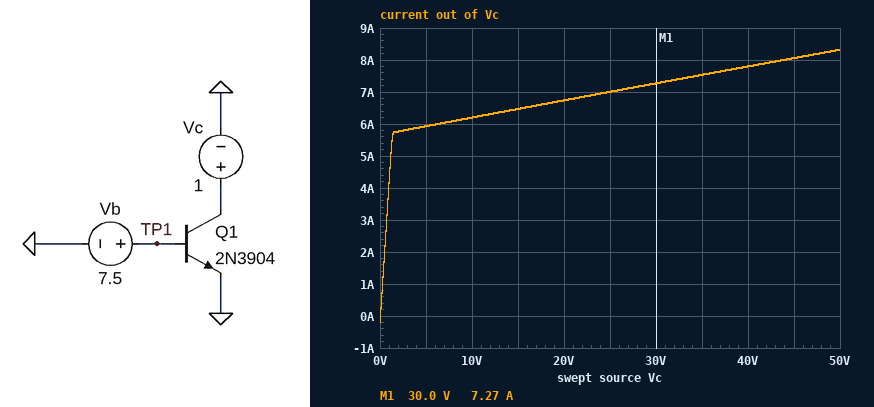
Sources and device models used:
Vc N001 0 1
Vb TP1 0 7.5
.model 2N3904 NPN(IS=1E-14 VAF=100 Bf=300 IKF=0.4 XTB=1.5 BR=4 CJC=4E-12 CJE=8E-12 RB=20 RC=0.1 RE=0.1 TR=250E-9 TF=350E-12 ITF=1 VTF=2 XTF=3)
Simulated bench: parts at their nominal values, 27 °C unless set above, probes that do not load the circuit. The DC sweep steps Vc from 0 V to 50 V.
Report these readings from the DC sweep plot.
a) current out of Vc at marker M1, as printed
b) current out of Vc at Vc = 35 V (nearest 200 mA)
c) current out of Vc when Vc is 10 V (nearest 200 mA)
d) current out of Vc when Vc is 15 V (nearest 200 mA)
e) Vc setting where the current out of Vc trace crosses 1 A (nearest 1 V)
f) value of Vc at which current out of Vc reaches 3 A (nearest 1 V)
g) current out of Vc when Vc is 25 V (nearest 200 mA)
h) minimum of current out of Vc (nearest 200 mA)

7.27 A
7.6 A
6.2 A
6.4 A
0 V
1 V
7.0 A
-200 mA
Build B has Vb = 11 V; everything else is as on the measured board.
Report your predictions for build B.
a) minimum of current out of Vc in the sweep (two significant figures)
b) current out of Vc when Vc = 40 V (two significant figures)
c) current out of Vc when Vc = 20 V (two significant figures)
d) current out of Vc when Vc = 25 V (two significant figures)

-290 mA
9.8 A
8.5 A
8.8 A
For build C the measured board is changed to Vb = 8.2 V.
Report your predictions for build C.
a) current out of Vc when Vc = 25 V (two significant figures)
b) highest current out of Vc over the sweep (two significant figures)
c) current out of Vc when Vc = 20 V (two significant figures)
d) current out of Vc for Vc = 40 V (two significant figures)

7.4 A
8.8 A
7.1 A
8.2 A
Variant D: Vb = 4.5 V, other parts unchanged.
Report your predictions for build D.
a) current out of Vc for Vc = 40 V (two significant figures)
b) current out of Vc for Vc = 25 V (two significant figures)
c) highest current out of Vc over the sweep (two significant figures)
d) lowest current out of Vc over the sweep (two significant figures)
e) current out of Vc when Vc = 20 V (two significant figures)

5.6 A
5.0 A
5.9 A
-110 mA
4.8 A
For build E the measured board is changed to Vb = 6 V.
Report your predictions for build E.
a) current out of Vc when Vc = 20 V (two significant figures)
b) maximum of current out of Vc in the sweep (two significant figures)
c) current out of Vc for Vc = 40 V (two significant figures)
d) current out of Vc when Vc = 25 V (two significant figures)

5.9 A
7.2 A
6.8 A
6.1 A
